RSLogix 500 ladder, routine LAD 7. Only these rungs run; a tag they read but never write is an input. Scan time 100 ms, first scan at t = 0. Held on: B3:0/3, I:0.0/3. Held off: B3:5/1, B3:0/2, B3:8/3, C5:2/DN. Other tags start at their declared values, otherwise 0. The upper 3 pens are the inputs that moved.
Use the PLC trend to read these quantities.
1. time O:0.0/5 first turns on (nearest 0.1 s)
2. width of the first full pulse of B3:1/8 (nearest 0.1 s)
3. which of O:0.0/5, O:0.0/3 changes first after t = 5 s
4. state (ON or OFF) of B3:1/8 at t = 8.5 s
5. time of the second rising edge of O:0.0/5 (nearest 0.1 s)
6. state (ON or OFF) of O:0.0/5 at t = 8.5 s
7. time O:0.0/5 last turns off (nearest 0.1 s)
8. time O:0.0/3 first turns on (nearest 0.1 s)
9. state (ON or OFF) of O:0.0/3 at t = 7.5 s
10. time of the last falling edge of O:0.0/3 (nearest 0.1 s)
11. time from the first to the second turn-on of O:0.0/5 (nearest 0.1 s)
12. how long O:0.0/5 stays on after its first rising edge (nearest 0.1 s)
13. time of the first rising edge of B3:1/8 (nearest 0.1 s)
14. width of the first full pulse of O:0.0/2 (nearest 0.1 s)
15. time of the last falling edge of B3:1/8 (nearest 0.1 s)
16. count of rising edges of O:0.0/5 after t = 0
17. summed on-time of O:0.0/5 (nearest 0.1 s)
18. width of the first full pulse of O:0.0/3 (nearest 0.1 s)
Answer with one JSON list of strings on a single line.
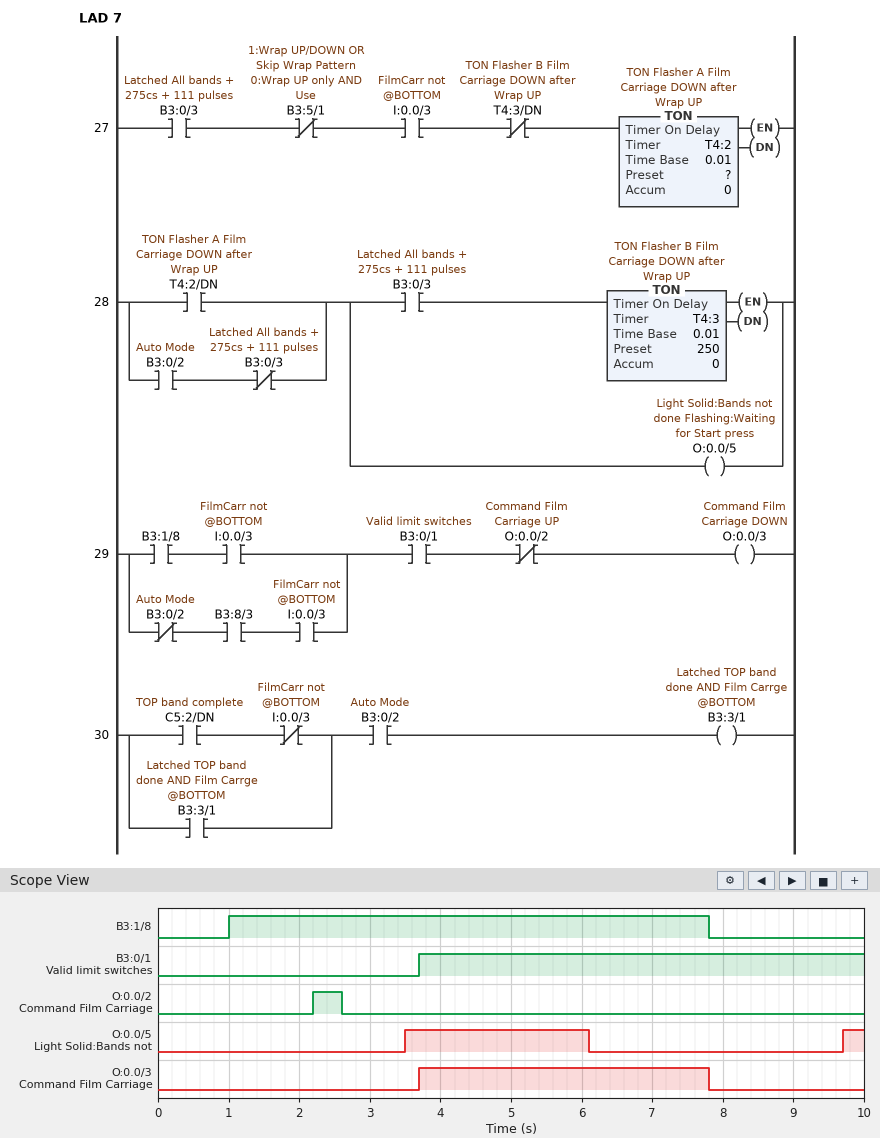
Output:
["3.5 s", "6.8 s", "O:0.0/5", "OFF", "9.7 s", "OFF", "6.1 s", "3.7 s", "ON", "7.8 s", "6.2 s", "2.6 s", "1.0 s", "0.4 s", "7.8 s", "2", "2.9 s", "4.1 s"]
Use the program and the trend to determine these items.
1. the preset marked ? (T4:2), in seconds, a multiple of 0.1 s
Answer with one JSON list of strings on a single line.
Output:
["3.5 s"]
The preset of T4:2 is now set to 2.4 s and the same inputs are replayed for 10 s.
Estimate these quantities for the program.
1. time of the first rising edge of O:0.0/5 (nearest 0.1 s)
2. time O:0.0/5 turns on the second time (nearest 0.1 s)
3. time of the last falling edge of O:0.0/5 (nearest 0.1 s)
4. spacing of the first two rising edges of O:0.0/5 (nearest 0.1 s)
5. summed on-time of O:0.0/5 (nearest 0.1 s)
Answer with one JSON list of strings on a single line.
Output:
["2.4 s", "7.5 s", "5.0 s", "5.1 s", "5.1 s"]
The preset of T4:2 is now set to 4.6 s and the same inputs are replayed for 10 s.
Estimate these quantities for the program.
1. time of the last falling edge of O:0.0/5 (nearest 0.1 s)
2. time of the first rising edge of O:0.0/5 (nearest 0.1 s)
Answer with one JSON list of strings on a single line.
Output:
["7.2 s", "4.6 s"]
